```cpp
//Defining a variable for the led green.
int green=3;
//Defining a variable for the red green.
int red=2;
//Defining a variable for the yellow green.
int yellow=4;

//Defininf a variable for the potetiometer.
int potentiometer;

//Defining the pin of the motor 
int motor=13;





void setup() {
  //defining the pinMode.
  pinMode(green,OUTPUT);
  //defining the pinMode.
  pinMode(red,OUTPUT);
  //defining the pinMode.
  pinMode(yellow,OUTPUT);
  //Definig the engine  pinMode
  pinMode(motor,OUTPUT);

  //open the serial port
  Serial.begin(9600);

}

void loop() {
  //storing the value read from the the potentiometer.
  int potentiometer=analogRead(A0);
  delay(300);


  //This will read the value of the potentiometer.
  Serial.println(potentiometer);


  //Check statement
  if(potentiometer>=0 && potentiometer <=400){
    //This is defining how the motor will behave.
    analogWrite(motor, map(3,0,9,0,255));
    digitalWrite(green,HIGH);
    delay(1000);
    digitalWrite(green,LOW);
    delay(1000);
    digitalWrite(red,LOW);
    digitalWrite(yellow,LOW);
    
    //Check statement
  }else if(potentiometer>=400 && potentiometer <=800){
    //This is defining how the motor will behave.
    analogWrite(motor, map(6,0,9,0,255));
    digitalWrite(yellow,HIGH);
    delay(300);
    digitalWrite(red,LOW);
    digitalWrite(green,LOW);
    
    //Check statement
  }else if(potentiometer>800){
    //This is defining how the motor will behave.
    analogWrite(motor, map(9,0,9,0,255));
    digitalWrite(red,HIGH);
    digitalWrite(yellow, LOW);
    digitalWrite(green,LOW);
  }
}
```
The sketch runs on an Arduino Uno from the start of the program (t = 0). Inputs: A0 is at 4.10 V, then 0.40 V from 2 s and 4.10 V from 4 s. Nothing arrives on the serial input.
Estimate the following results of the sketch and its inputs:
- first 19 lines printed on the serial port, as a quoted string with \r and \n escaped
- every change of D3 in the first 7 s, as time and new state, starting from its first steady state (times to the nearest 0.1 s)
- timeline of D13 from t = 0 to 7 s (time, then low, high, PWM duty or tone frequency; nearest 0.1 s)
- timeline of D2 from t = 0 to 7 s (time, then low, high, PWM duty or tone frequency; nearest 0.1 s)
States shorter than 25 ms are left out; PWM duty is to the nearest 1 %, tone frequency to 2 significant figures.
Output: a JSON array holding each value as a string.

["\"839\\r\\n839\\r\\n839\\r\\n839\\r\\n839\\r\\n839\\r\\n839\\r\\n81\\r\\n839\\r\\n839\\r\\n839\\r\\n839\\r\\n839\\r\\n839\\r\\n839\\r\\n839\\r\\n839\\r\\n839\\r\\n839\\r\\n\"", "0 s low; 2.4 s high; 3.4 s low", "0 s low; 0.3 s high; 2.4 s low; 4.7 s high", "0 s low; 0.3 s high; 4.4 s low; 4.7 s high"]
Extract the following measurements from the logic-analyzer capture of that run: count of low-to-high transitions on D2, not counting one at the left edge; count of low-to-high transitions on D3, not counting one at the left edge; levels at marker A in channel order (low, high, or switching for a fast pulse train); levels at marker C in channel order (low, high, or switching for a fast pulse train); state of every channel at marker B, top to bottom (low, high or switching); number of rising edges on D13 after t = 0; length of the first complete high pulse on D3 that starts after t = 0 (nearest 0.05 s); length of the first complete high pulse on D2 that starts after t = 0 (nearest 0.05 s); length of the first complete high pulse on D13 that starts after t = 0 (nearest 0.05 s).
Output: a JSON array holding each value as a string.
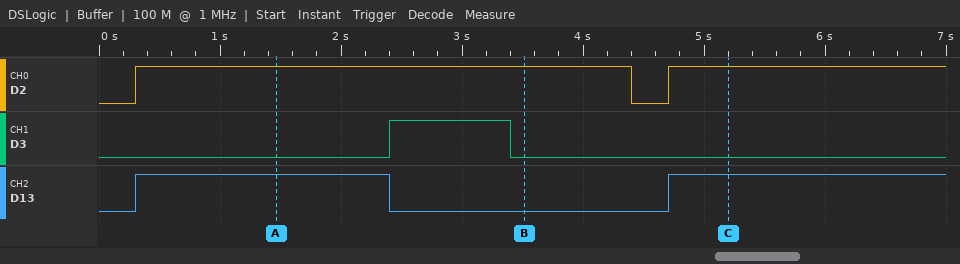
["2", "1", "D2 high, D3 low, D13 high", "D2 high, D3 low, D13 high", "D2 high, D3 low, D13 low", "2", "1.00 s", "4.10 s", "2.10 s"]
